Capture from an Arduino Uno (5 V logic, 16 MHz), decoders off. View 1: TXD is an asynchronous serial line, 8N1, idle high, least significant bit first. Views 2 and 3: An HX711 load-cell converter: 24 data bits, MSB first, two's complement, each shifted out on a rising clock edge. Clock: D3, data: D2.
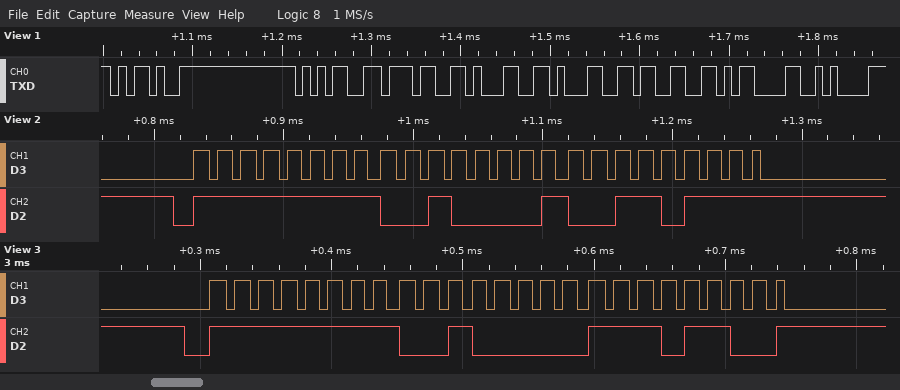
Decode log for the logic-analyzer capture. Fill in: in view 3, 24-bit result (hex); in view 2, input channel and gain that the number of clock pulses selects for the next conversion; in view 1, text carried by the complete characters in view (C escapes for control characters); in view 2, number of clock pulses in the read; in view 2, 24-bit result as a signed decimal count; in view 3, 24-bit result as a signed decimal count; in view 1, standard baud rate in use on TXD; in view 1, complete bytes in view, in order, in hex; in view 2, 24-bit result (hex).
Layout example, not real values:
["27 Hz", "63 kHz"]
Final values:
["0xFF20EC", "channel A, gain 128", "\"-57113\\r\\n\"", "25", "-57033", "-57108", "115200 baud", "0x2D 0x35 0x37 0x31 0x31 0x33 0x0D 0x0A", "0xFF2137"]
